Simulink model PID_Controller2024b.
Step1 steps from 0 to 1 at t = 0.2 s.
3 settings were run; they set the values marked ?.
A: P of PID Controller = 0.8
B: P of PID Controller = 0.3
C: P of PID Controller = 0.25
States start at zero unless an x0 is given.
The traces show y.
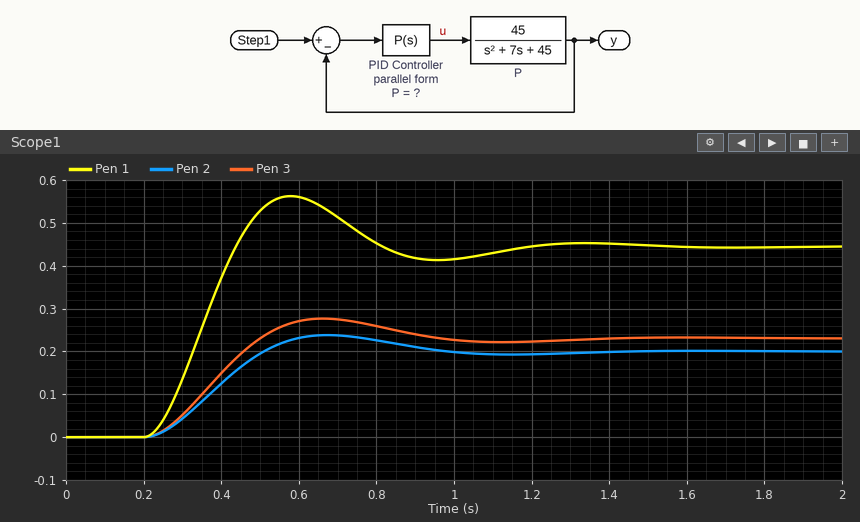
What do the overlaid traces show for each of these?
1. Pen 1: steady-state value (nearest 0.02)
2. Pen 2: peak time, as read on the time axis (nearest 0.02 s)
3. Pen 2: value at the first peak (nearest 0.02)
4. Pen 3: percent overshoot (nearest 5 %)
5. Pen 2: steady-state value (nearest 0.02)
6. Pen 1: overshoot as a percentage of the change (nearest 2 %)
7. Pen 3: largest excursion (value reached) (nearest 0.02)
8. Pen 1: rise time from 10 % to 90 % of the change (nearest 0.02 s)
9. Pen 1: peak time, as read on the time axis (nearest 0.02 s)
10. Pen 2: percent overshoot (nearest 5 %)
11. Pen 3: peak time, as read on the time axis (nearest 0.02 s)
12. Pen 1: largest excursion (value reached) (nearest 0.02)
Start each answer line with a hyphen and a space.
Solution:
- 0.44
- 0.68 s
- 0.24
- 20 %
- 0.20
- 26 %
- 0.28
- 0.16 s
- 0.58 s
- 20 %
- 0.66 s
- 0.56
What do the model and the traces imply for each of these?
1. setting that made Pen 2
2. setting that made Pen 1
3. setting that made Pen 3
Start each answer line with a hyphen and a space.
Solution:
- C
- A
- B
